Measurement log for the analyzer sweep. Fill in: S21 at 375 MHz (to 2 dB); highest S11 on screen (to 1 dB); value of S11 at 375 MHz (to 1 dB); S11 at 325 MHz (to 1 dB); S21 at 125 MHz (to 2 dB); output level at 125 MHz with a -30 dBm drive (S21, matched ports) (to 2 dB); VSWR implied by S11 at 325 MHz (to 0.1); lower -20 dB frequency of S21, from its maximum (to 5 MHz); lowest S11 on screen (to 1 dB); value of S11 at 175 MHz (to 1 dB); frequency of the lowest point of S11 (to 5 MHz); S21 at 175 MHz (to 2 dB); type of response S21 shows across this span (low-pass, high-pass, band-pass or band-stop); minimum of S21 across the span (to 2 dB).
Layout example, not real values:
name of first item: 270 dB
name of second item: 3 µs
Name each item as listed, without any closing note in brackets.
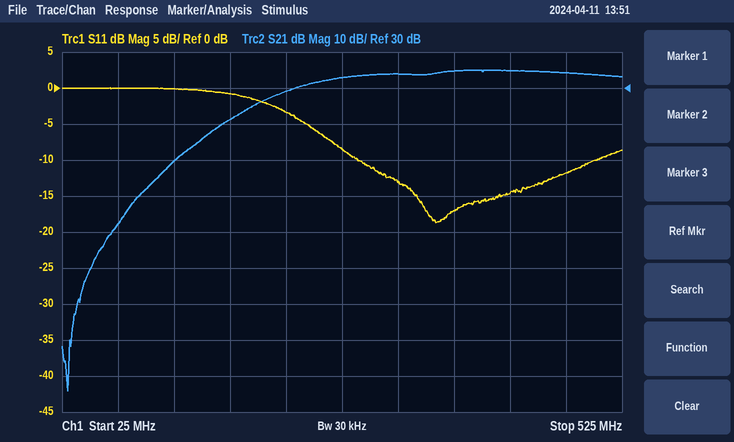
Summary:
S21 at 375 MHz: 34 dB
highest S11 on screen: 0 dB
value of S11 at 375 MHz: -17 dB
S11 at 325 MHz: -13 dB
S21 at 125 MHz: 10 dB
output level at 125 MHz with a -30 dBm drive (S21, matched ports): -20 dBm
VSWR implied by S11 at 325 MHz: 1.6
lower -20 dB frequency of S21, from its maximum: 145 MHz
lowest S11 on screen: -19 dB
value of S11 at 175 MHz: -1 dB
frequency of the lowest point of S11: 360 MHz
S21 at 175 MHz: 22 dB
type of response S21 shows across this span: high-pass
minimum of S21 across the span: -54 dB
